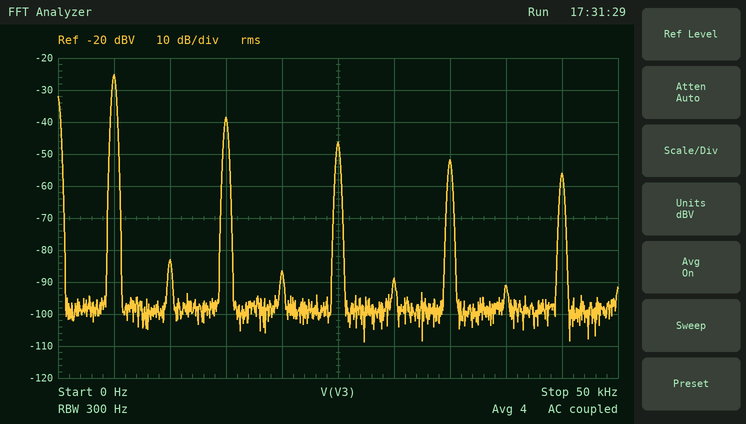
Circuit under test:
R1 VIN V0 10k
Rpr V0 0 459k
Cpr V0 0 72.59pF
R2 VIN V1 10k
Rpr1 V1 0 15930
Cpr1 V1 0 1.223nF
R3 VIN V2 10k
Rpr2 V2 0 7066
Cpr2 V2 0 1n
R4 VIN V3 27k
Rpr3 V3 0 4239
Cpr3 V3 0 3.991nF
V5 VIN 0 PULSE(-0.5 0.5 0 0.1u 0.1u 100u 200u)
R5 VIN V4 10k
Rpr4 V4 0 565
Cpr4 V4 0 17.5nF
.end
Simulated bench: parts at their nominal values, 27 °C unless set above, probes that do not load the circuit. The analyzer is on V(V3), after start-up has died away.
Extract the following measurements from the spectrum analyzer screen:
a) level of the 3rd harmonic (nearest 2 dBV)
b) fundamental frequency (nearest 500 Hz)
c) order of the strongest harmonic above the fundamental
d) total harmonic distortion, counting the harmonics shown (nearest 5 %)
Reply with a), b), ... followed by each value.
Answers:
a) -38 dBV
b) 5.0 kHz
c) 3
d) 25 %
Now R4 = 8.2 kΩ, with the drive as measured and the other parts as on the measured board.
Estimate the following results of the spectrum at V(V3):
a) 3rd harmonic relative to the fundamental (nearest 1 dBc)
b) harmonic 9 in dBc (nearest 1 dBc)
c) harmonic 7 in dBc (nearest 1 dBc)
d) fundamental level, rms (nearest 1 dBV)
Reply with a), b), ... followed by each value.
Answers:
a) -12 dBc
b) -29 dBc
c) -25 dBc
d) -17 dBV
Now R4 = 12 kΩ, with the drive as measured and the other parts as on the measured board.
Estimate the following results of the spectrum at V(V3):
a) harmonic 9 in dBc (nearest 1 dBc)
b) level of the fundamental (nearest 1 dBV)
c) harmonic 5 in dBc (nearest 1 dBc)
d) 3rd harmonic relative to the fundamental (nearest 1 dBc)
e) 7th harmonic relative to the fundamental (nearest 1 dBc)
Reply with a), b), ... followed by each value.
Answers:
a) -30 dBc
b) -19 dBV
c) -20 dBc
d) -13 dBc
e) -26 dBc
